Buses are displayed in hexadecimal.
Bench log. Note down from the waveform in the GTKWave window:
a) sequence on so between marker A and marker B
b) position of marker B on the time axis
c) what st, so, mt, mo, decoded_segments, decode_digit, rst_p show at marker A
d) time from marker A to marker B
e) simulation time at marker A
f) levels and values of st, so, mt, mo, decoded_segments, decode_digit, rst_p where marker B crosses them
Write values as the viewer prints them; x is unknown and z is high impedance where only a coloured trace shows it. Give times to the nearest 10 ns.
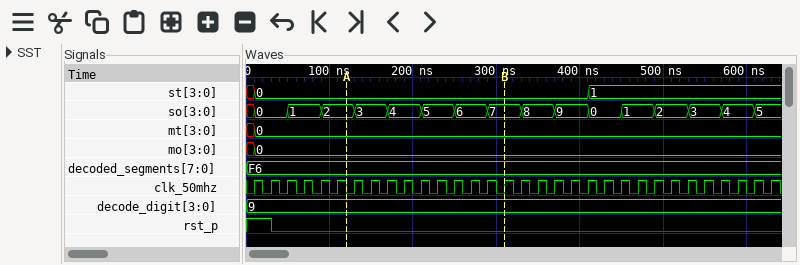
2, 3, 4, 5, 6, 7
310 ns
st=0, so=2, mt=0, mo=0, decoded_segments=F6, decode_digit=9, rst_p=0
190 ns
120 ns
st=0, so=7, mt=0, mo=0, decoded_segments=F6, decode_digit=9, rst_p=0
